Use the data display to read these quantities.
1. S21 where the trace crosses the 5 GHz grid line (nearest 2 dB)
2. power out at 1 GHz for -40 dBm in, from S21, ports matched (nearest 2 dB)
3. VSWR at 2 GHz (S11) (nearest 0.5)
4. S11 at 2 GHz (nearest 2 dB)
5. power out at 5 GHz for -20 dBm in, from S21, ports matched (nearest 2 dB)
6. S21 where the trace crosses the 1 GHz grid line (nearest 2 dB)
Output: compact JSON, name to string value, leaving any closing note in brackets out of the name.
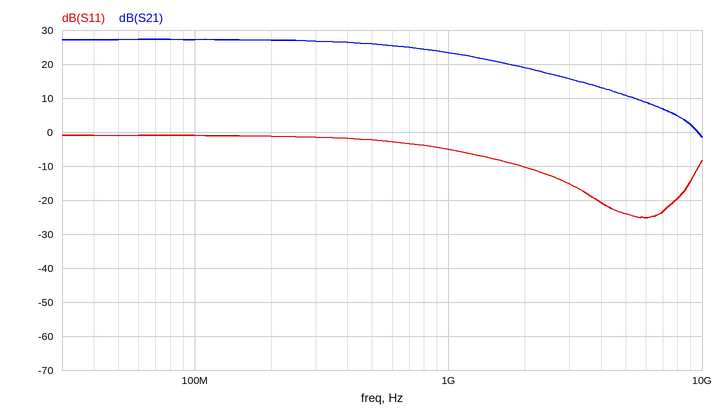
{"S21 where the trace crosses the 5 GHz grid line": "10 dB", "power out at 1 GHz for -40 dBm in, from S21, ports matched": "-16 dBm", "VSWR at 2 GHz (S11)": "2.0", "S11 at 2 GHz": "-10 dB", "power out at 5 GHz for -20 dBm in, from S21, ports matched": "-10 dBm", "S21 where the trace crosses the 1 GHz grid line": "24 dB"}
